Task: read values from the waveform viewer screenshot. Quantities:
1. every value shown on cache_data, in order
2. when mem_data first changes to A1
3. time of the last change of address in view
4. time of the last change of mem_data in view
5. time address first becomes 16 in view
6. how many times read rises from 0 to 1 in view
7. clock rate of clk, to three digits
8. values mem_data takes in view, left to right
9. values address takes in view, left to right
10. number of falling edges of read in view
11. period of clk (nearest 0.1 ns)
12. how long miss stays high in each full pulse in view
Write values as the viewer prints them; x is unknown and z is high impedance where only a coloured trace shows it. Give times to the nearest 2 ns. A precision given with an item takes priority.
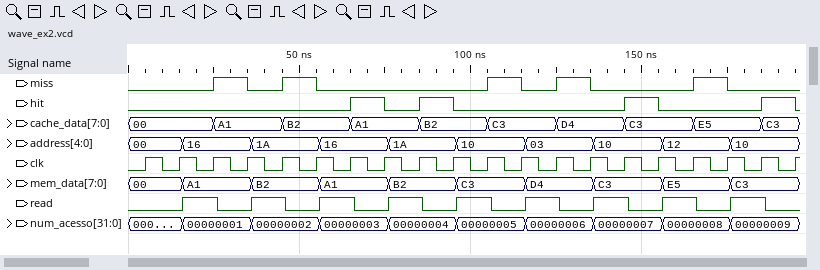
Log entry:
00, A1, B2, A1, B2, C3, D4, C3, E5, C3
16 ns
176 ns
176 ns
16 ns
9
100 MHz
00, A1, B2, A1, B2, C3, D4, C3, E5, C3
00, 16, 1A, 16, 1A, 10, 03, 10, 12, 10
9
10 ns
10 ns, 10 ns, 10 ns, 10 ns, 10 ns
